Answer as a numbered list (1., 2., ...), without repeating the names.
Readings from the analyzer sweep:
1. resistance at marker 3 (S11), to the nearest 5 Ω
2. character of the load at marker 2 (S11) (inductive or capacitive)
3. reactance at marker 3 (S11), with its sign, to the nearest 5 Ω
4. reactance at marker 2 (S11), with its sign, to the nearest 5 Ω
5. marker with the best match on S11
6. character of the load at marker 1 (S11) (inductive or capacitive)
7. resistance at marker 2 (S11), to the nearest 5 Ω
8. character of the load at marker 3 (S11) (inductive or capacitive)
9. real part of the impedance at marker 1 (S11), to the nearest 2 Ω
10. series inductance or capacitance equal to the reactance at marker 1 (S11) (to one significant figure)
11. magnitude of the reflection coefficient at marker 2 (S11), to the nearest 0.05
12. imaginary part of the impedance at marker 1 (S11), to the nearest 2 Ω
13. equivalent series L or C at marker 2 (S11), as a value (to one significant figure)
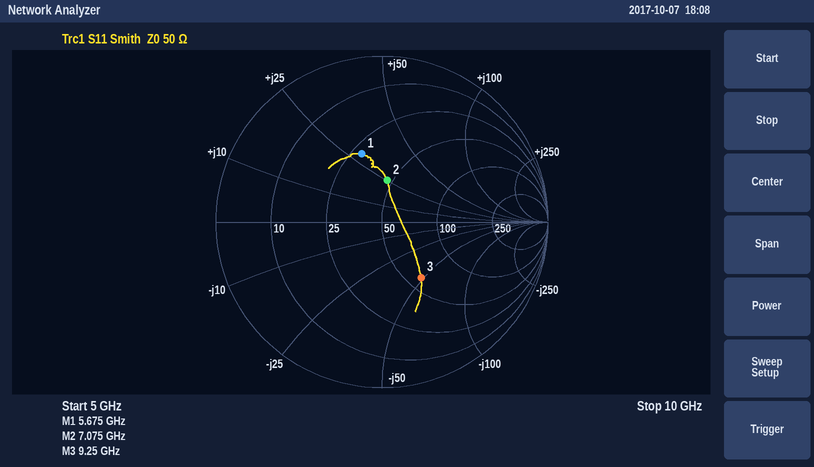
1. 60 Ω
2. inductive
3. -50 Ω
4. +25 Ω
5. marker 2
6. inductive
7. 45 Ω
8. capacitive
9. 28 Ω
10. 800 pH
11. 0.25
12. +28 Ω
13. 600 pH
